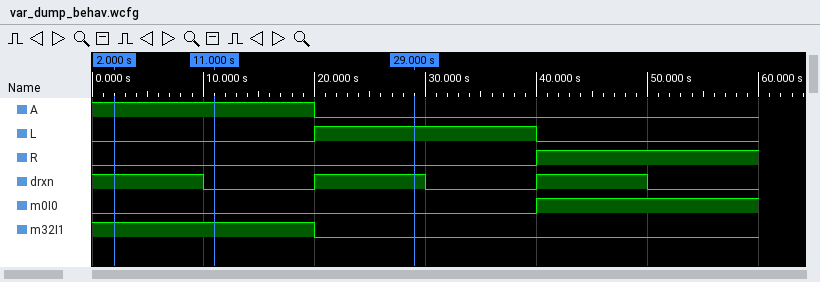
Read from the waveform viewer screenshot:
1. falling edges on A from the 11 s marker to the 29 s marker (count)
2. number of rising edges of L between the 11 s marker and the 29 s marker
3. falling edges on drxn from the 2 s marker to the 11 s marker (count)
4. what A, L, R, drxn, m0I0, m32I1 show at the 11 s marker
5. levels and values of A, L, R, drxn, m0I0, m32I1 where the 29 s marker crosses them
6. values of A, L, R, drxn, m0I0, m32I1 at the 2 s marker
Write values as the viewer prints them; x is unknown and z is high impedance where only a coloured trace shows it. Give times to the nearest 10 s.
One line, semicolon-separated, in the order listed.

1; 1; 1; A=1, L=0, R=0, drxn=0, m0I0=0, m32I1=1; A=0, L=1, R=0, drxn=1, m0I0=0, m32I1=0; A=1, L=0, R=0, drxn=1, m0I0=0, m32I1=1
